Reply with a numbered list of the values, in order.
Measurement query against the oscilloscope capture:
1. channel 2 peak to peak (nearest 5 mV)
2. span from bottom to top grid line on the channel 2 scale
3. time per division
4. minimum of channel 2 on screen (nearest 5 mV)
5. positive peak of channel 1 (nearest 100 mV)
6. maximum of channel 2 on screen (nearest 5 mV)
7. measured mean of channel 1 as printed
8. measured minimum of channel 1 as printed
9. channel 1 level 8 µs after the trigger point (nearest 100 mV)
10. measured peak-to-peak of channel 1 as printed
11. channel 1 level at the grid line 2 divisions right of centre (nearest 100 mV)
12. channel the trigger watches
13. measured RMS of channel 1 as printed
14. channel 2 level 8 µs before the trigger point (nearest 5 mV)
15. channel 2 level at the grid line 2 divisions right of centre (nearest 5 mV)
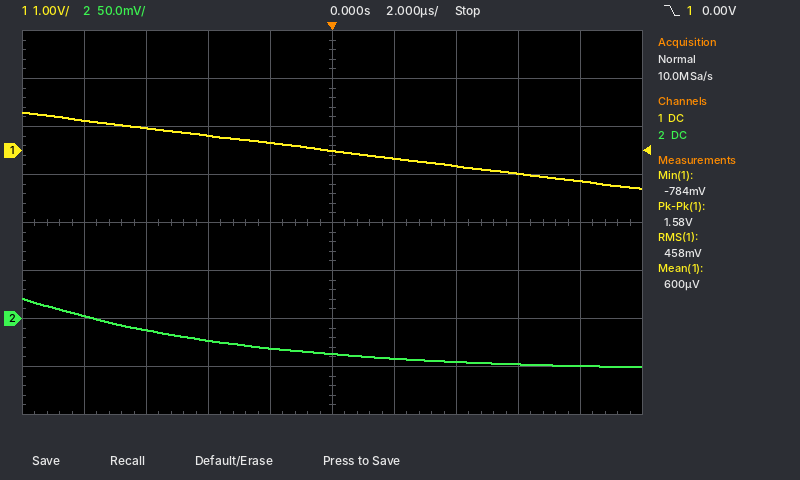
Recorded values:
1. 70 mV
2. 400 mV
3. 2 µs
4. -50 mV
5. 800 mV
6. 20 mV
7. 600 µV
8. -784 mV
9. -600 mV
10. 1.58 V
11. -300 mV
12. channel 1
13. 458 mV
14. 5 mV
15. -45 mV
